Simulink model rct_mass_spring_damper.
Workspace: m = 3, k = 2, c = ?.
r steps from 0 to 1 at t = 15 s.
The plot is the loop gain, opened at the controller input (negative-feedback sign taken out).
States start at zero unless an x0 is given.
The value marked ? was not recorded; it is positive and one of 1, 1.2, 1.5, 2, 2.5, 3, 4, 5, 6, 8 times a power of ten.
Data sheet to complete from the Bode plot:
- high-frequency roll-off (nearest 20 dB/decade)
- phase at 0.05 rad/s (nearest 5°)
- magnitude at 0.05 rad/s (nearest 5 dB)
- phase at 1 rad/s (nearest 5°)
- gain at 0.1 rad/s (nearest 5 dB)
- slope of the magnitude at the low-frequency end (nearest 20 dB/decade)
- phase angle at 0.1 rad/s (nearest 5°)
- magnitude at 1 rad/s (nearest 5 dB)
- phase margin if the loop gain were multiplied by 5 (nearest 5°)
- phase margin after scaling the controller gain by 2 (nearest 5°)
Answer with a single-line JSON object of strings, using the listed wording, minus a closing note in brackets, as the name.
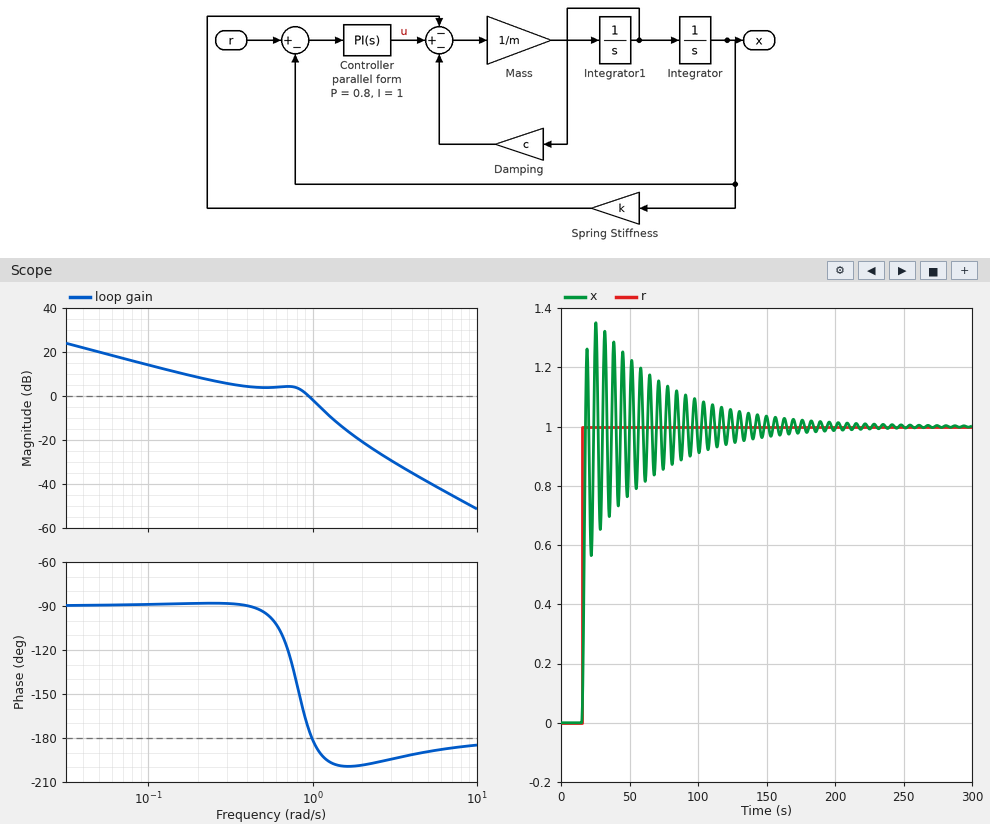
{"high-frequency roll-off": "-40 dB/decade", "phase at 0.05 rad/s": "-90°", "magnitude at 0.05 rad/s": "20 dB", "phase at 1 rad/s": "-180°", "gain at 0.1 rad/s": "15 dB", "slope of the magnitude at the low-frequency end": "-20 dB/decade", "phase angle at 0.1 rad/s": "-90°", "magnitude at 1 rad/s": "0 dB", "phase margin if the loop gain were multiplied by 5": "-20°", "phase margin after scaling the controller gain by 2": "-10°"}
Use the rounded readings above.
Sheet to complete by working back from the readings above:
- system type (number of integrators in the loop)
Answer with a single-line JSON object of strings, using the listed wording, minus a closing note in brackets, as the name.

{"system type": "1"}
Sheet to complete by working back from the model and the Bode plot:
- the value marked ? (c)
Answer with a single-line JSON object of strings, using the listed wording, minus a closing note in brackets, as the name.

{"the value marked ?": "1.2"}
